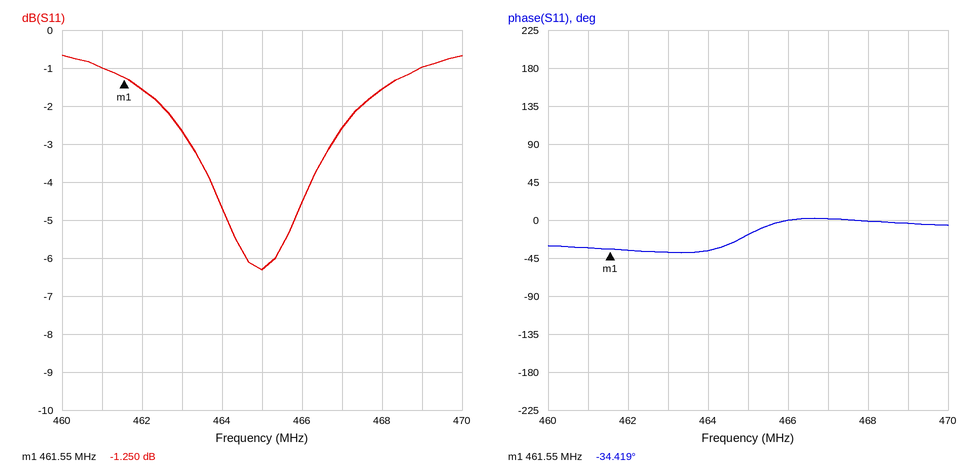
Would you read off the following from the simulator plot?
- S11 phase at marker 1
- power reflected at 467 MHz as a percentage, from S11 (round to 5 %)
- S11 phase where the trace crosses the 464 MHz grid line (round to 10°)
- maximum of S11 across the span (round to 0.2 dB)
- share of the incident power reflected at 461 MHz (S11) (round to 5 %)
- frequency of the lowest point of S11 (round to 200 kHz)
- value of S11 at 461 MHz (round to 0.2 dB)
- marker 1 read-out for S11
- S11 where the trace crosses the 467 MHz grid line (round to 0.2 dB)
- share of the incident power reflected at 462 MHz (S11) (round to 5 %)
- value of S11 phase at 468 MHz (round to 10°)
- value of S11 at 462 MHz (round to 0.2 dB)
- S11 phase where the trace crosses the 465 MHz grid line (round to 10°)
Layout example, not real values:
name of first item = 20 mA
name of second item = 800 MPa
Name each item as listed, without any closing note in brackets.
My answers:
S11 phase at marker 1 = -34.419°
power reflected at 467 MHz as a percentage, from S11 = 55 %
S11 phase where the trace crosses the 464 MHz grid line = -40°
maximum of S11 across the span = -0.6 dB
share of the incident power reflected at 461 MHz (S11) = 80 %
frequency of the lowest point of S11 = 465.0 MHz
value of S11 at 461 MHz = -1.0 dB
marker 1 read-out for S11 = -1.250 dB
S11 where the trace crosses the 467 MHz grid line = -2.6 dB
share of the incident power reflected at 462 MHz (S11) = 70 %
value of S11 phase at 468 MHz = 0°
value of S11 at 462 MHz = -1.6 dB
S11 phase where the trace crosses the 465 MHz grid line = -20°
